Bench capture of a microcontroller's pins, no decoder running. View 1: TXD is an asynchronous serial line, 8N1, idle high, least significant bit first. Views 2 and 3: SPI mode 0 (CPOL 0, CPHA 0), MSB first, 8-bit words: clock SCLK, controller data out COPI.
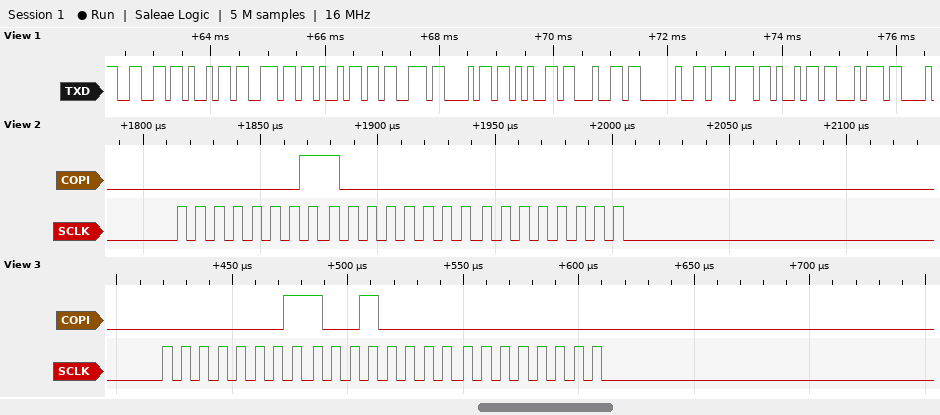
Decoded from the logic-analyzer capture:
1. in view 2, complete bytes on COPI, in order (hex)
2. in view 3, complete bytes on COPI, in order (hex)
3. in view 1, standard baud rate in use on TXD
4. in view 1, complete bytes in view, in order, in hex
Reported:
01 80 00
01 90 00
9600 baud
66 69 6E 69 73 68 65 64 20 77 69 74
